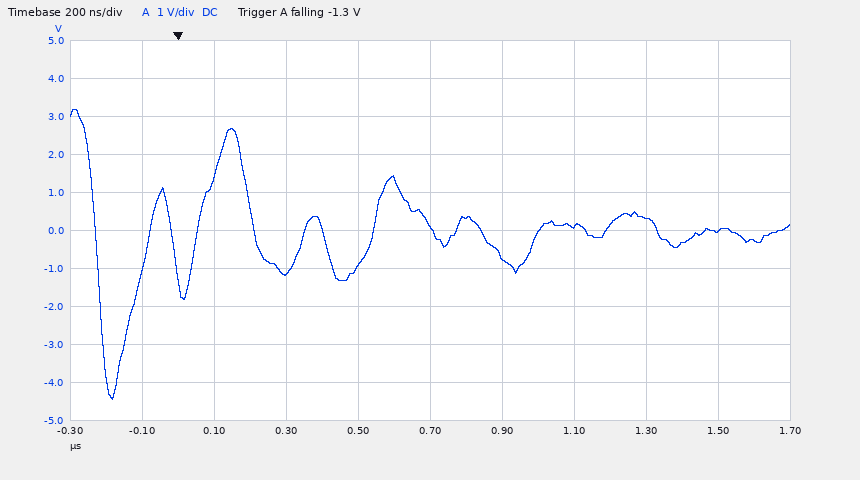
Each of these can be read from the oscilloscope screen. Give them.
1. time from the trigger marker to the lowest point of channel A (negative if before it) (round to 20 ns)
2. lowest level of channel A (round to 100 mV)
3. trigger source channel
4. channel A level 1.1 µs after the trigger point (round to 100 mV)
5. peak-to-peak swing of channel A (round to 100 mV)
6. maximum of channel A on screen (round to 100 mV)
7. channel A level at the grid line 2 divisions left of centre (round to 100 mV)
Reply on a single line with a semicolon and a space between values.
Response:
-180 ns; -4.4 V; channel A; 100 mV; 7.6 V; 3.2 V; -1.1 V
